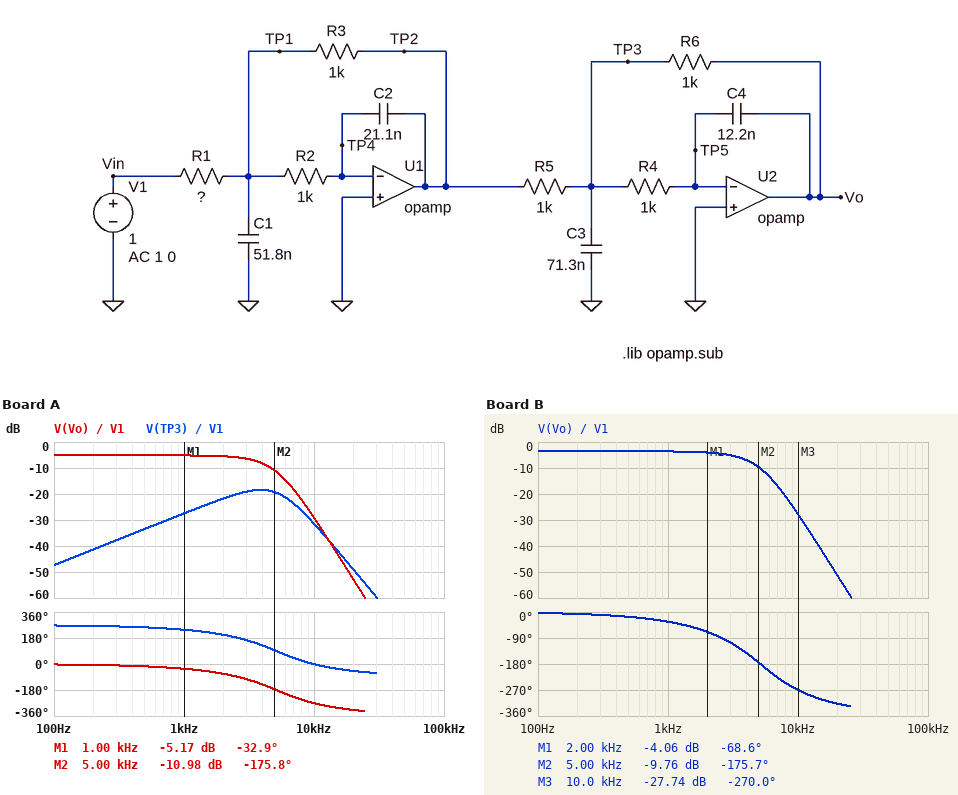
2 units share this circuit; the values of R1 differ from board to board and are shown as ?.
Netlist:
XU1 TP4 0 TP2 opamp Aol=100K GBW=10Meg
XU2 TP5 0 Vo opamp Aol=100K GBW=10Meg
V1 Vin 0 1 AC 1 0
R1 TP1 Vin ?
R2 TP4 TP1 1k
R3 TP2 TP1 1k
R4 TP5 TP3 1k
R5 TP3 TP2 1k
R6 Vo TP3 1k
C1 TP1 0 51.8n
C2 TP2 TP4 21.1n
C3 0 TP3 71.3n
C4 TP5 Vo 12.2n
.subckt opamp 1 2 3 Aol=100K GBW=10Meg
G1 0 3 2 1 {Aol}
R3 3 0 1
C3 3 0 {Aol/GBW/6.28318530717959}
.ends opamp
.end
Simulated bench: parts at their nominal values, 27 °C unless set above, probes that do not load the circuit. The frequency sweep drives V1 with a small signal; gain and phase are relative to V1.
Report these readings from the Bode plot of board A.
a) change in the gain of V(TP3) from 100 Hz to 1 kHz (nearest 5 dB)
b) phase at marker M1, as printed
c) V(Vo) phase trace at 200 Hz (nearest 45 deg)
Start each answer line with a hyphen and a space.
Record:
- 20 dB
- -32.9 deg
- 0 deg
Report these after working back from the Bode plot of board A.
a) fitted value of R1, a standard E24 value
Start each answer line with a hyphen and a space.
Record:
- 1.8 kΩ
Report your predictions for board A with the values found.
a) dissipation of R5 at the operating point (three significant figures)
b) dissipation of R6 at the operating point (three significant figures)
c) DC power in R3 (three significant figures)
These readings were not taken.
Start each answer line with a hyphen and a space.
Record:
- 309 µW
- 309 µW
- 309 µW
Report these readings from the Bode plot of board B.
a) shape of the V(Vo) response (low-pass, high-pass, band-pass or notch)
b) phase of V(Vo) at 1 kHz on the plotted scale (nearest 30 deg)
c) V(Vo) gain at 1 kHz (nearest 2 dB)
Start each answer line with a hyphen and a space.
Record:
- low-pass
- -30 deg
- -4 dB
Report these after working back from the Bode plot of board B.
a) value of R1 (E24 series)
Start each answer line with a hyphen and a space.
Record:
- 1.5 kΩ
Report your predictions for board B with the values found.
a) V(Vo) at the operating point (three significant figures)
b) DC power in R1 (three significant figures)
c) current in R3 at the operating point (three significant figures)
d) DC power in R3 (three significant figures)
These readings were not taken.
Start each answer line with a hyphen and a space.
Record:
- 667 mV
- 667 µW
- 667 µA
- 444 µW
